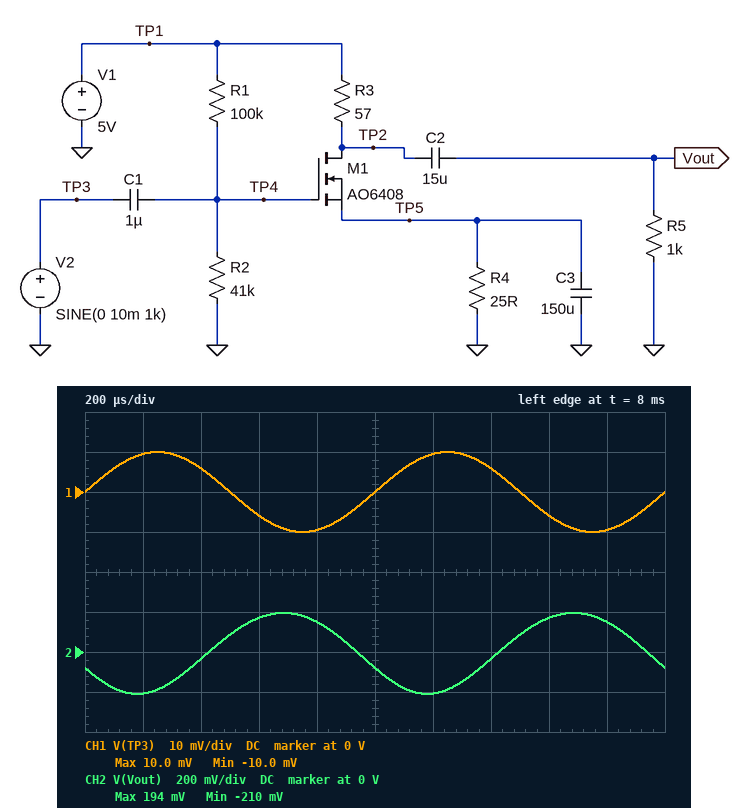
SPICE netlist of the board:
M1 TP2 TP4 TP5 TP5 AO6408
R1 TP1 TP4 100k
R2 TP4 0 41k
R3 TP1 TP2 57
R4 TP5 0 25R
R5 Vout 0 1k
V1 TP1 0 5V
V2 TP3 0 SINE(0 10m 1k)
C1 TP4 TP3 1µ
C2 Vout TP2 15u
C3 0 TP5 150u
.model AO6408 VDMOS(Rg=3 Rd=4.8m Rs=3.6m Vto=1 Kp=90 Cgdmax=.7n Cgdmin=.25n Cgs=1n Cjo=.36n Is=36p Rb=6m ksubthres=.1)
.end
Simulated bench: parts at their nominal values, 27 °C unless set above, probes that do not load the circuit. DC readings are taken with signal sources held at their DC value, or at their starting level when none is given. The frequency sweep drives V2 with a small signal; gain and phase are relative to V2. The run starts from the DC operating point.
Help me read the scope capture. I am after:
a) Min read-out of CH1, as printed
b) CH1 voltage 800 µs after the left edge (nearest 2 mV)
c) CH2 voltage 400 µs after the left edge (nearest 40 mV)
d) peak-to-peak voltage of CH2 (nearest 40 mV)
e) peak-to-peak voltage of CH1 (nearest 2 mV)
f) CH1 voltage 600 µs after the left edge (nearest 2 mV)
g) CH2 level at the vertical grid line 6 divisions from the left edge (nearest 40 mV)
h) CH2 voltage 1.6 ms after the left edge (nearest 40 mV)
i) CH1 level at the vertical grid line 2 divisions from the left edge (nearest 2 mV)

-10.0 mV
-10 mV
-40 mV
400 mV
20 mV
-6 mV
-200 mV
160 mV
6 mV
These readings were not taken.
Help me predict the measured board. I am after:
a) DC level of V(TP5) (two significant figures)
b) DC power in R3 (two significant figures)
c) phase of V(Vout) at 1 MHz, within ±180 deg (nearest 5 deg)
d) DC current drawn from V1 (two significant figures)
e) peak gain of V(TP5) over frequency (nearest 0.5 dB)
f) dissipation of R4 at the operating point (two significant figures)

590 mV
32 mW
160 deg
24 mA
-1.0 dB
14 mW
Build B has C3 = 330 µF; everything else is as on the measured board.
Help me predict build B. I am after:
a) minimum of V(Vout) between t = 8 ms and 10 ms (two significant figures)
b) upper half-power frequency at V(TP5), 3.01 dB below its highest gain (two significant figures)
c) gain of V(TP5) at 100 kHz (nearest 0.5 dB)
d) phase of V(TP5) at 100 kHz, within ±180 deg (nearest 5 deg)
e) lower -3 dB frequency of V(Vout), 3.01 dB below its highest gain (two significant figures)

-230 mV
230 Hz
-54.0 dB
-90 deg
220 Hz
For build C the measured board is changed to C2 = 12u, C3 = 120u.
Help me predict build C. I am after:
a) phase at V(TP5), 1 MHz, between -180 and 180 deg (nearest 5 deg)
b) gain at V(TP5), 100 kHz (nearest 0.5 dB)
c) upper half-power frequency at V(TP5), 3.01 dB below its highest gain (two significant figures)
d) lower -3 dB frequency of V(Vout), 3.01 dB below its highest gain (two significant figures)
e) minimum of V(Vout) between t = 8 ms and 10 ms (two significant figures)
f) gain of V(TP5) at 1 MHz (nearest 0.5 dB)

-100 deg
-45.0 dB
620 Hz
600 Hz
-200 mV
-65.5 dB
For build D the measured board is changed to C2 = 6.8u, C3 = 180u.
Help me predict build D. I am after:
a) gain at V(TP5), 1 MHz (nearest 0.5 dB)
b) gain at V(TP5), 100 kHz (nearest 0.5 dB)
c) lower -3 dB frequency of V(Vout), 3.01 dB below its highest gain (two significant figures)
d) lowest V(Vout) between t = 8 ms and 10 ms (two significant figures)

-69.0 dB
-48.5 dB
400 Hz
-220 mV
